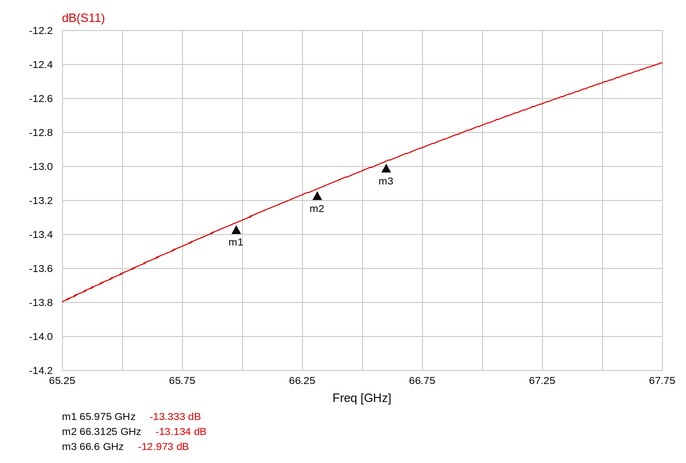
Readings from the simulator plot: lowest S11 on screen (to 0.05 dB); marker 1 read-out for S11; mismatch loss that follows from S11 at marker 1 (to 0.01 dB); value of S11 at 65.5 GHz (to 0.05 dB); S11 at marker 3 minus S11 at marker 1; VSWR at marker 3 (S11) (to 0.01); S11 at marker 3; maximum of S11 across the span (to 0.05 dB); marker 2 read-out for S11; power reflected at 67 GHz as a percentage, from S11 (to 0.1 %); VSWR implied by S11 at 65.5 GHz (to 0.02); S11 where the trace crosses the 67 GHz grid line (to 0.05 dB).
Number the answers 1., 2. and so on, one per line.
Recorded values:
1. -13.80 dB
2. -13.333 dB
3. 0.21 dB
4. -13.65 dB
5. 0.360 dB
6. 1.58
7. -12.973 dB
8. -12.40 dB
9. -13.134 dB
10. 5.3 %
11. 1.52
12. -12.75 dB
